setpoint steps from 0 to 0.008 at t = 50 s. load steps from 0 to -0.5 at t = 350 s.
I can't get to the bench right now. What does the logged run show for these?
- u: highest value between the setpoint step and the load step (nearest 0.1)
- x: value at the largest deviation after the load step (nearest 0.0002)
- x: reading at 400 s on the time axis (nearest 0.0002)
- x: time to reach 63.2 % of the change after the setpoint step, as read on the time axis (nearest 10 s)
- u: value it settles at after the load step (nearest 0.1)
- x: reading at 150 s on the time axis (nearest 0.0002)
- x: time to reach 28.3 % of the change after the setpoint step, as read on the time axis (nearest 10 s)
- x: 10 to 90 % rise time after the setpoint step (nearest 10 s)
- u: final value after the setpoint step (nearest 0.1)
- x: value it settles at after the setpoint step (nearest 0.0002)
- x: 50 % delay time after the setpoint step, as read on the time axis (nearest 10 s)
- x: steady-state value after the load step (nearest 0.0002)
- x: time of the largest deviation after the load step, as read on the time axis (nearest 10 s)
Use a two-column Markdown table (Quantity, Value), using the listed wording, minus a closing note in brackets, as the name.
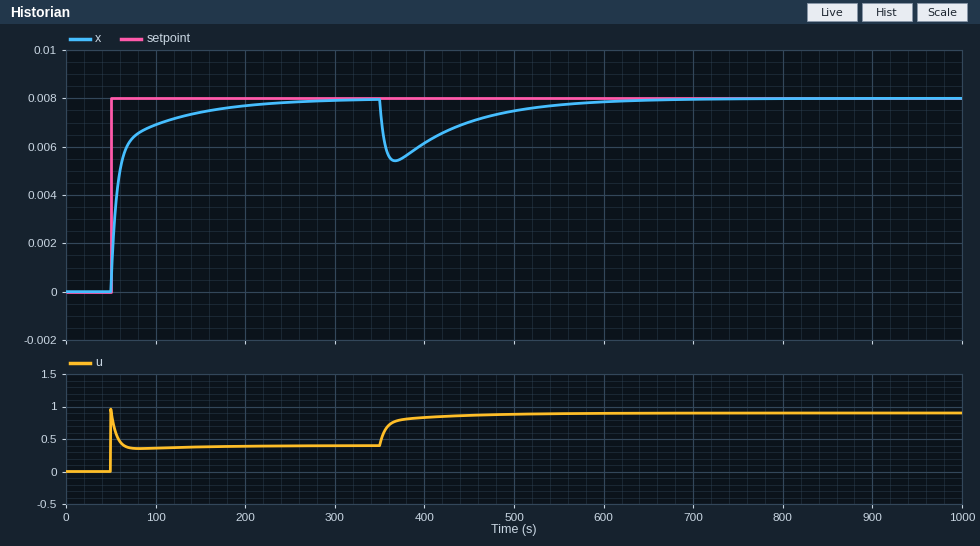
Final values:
| Quantity | Value |
|---|---|
| u: highest value between the setpoint step and the load step | 1.0 |
| x: value at the largest deviation after the load step | 0.0054 |
| x: reading at 400 s on the time axis | 0.0062 |
| x: time to reach 63.2 % of the change after the setpoint step, as read on the time axis | 60 s |
| u: value it settles at after the load step | 0.9 |
| x: reading at 150 s on the time axis | 0.0074 |
| x: time to reach 28.3 % of the change after the setpoint step, as read on the time axis | 50 s |
| x: 10 to 90 % rise time after the setpoint step | 70 s |
| u: final value after the setpoint step | 0.4 |
| x: value it settles at after the setpoint step | 0.0080 |
| x: 50 % delay time after the setpoint step, as read on the time axis | 60 s |
| x: steady-state value after the load step | 0.0080 |
| x: time of the largest deviation after the load step, as read on the time axis | 370 s |
